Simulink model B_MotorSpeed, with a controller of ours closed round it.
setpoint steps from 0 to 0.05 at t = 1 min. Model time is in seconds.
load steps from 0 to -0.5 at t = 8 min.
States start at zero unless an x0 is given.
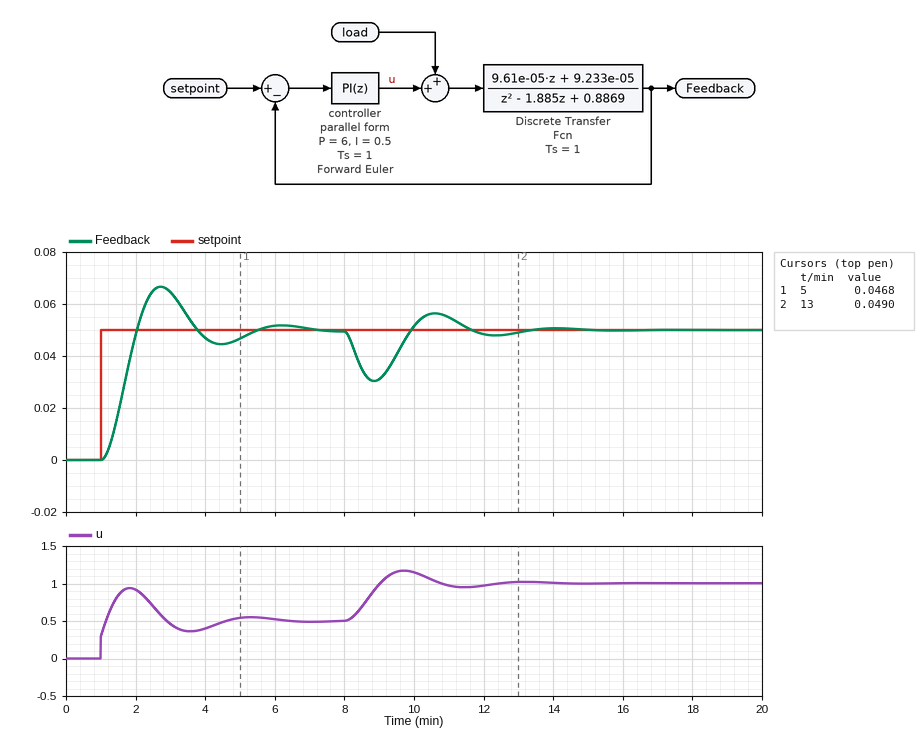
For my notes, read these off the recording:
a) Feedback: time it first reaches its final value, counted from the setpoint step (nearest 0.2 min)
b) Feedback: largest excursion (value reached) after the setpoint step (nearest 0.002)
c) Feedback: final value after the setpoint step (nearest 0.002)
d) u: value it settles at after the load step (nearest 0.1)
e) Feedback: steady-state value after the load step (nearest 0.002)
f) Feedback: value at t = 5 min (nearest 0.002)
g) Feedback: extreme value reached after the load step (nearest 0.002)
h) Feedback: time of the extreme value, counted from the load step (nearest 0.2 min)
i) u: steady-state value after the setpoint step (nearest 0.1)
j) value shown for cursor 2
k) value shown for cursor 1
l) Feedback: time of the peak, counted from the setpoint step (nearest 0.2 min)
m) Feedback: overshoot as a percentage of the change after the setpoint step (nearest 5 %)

1.0 min
0.066
0.050
1.0
0.050
0.046
0.030
0.8 min
0.5
0.0490
0.0468
1.8 min
35 %
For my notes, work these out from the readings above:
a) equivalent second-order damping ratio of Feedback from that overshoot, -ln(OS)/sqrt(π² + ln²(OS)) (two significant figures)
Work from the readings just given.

0.32
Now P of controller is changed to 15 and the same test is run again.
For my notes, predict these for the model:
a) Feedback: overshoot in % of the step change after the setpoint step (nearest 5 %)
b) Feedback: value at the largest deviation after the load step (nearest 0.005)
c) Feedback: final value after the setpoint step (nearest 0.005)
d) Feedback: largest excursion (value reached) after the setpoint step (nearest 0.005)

15 %
0.035
0.050
0.055
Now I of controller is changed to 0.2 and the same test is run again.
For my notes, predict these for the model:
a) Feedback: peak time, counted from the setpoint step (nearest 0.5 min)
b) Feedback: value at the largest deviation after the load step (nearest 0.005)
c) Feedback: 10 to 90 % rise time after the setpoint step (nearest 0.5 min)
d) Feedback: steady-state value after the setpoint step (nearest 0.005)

3.0 min
0.025
1.5 min
0.050
